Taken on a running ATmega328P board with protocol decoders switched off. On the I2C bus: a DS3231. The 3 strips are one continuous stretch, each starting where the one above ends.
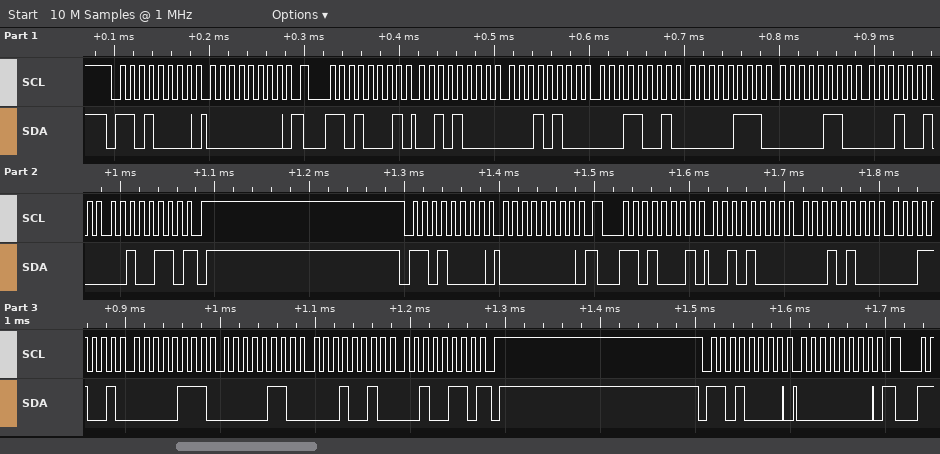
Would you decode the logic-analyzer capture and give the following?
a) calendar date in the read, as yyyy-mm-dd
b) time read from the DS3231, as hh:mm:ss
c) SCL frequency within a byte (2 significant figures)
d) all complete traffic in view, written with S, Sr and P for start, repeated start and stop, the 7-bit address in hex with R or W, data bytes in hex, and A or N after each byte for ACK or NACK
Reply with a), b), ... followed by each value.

a) 2026-12-06
b) 19:14:28
c) 100 kHz
d) S 68W A 00 A Sr 68R A 28 A 14 A 19 A 07 A 06 A 12 A 26 N P S 68W A 00 A Sr 68R A 28 A 14 A 19 A 07 A 06 A 12 A 26 N P S 68W A 00 A
